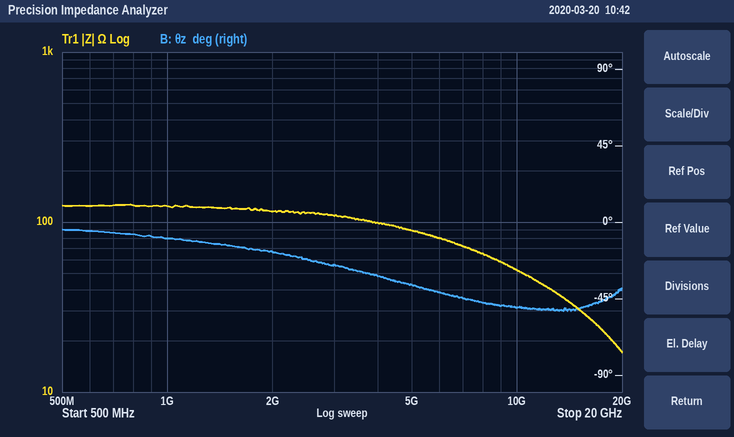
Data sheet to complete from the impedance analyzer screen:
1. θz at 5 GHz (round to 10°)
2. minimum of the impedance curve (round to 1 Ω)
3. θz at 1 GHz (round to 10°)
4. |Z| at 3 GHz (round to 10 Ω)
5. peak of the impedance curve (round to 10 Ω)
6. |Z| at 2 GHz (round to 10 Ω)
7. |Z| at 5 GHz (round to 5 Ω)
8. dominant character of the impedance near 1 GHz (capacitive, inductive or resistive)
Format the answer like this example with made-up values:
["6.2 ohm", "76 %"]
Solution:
["-40°", "17 Ω", "-10°", "110 Ω", "130 Ω", "120 Ω", "90 Ω", "resistive"]
